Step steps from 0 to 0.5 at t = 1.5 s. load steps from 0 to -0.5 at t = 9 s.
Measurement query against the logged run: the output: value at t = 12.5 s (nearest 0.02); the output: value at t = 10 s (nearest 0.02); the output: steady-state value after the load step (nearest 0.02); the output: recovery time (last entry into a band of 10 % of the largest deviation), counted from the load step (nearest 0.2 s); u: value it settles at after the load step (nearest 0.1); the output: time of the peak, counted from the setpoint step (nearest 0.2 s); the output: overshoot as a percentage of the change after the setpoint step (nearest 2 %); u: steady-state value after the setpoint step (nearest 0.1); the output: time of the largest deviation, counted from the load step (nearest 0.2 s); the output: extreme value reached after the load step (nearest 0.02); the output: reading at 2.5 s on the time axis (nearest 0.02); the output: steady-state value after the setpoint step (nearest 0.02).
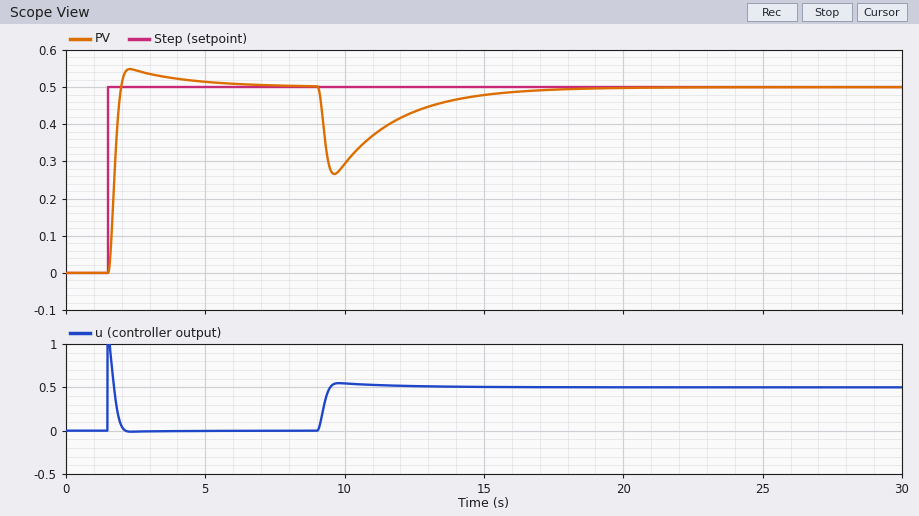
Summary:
0.44
0.30
0.50
5.8 s
0.5
0.8 s
10 %
0.0
0.6 s
0.26
0.54
0.50
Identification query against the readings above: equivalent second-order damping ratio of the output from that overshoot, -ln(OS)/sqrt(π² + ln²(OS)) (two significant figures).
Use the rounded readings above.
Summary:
0.59
